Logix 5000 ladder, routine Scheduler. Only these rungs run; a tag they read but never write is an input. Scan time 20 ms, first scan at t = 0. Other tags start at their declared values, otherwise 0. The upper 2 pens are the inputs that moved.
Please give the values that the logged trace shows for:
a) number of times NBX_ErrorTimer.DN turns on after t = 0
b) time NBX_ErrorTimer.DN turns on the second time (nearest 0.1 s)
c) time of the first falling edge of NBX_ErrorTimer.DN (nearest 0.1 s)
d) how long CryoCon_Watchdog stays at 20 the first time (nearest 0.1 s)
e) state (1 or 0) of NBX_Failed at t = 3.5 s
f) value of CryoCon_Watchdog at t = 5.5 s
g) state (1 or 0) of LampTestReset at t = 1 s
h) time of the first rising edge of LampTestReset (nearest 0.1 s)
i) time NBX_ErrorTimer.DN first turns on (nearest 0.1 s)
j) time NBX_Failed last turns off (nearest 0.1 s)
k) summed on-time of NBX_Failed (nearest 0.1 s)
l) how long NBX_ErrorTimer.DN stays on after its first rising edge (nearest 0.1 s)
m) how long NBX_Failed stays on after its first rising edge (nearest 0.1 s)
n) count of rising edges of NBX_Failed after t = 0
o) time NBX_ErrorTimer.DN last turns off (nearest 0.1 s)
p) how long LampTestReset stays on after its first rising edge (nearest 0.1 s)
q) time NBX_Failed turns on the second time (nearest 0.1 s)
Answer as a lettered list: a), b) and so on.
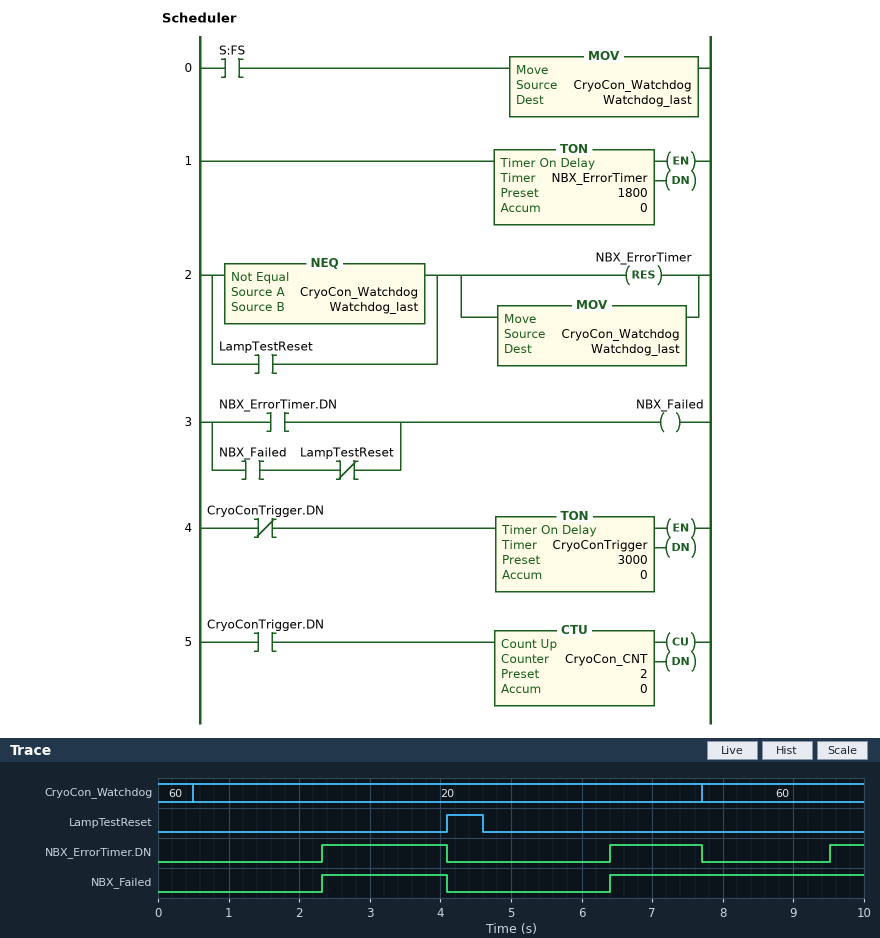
a) 3
b) 6.4 s
c) 4.1 s
d) 7.2 s
e) 1
f) 20
g) 0
h) 4.1 s
i) 2.3 s
j) 4.1 s
k) 5.4 s
l) 1.8 s
m) 1.8 s
n) 2
o) 7.7 s
p) 0.5 s
q) 6.4 s
